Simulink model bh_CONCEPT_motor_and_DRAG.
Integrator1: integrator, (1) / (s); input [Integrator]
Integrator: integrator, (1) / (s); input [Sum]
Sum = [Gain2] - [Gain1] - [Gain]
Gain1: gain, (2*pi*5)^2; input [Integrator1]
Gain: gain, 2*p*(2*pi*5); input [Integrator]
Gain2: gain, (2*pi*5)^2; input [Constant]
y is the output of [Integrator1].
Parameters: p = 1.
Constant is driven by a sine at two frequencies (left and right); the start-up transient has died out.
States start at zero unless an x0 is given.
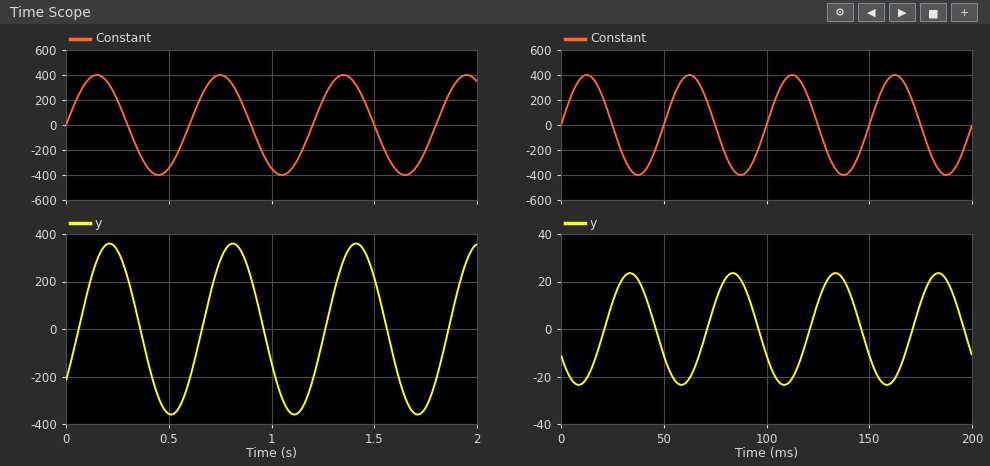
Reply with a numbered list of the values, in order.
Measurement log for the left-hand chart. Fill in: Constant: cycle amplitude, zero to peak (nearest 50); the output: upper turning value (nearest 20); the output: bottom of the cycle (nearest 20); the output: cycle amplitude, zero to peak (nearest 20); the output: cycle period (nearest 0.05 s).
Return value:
1. 400
2. 360
3. -360
4. 360
5. 0.60 s
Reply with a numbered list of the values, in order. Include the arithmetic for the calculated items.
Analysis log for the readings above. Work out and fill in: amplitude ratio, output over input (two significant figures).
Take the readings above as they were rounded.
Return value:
1. 360 / 400 = 0.90
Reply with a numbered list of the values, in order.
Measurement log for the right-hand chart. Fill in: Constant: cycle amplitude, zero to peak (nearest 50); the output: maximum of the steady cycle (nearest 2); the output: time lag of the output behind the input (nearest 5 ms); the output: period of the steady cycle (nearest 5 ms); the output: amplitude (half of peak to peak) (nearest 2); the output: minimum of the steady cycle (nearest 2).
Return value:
1. 400
2. 24
3. 20 ms
4. 50 ms
5. 24
6. -24
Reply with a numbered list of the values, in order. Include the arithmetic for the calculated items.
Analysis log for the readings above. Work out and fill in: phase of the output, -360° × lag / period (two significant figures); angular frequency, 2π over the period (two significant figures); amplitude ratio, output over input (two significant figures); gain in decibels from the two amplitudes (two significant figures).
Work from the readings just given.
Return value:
1. -360 × 20 / 50 = -140°
2. 2π / 50 = 0.13 rad/ms
3. 24 / 400 = 0.060
4. 20 log10(24 / 400) = -24 dB
